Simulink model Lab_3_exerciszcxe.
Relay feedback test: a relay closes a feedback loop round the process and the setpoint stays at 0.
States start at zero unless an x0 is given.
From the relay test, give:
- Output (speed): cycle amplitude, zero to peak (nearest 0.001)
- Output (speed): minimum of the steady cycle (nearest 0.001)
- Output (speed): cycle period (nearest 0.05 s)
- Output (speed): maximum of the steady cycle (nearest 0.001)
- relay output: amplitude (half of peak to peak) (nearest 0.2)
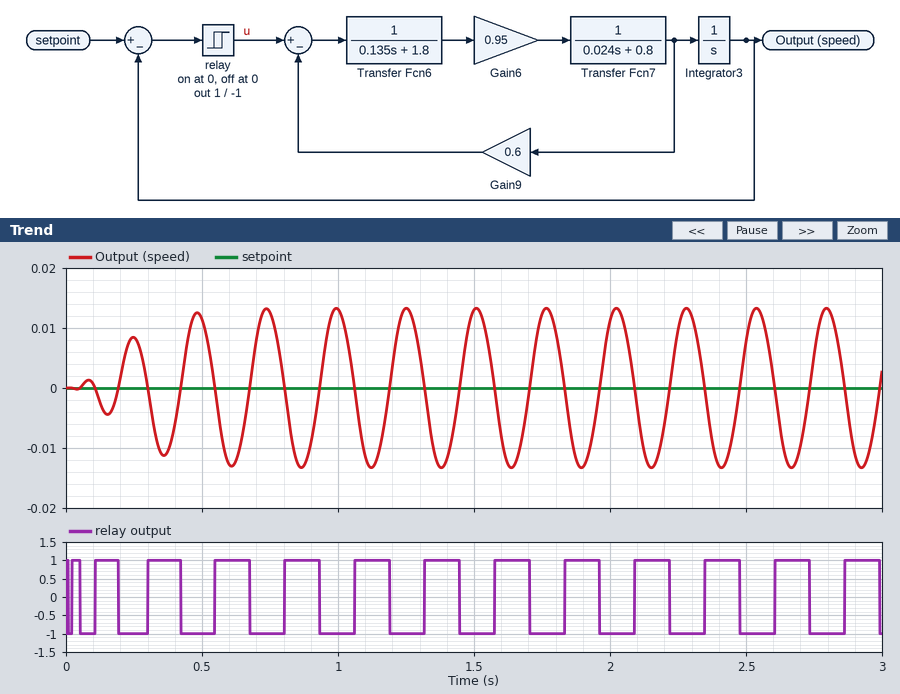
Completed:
0.013
-0.013
0.25 s
0.013
1.0
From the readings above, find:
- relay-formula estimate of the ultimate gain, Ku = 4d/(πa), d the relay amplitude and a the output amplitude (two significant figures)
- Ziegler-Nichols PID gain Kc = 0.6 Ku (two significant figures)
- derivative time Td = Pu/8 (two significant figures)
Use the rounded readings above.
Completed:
98
59
0.031 s
